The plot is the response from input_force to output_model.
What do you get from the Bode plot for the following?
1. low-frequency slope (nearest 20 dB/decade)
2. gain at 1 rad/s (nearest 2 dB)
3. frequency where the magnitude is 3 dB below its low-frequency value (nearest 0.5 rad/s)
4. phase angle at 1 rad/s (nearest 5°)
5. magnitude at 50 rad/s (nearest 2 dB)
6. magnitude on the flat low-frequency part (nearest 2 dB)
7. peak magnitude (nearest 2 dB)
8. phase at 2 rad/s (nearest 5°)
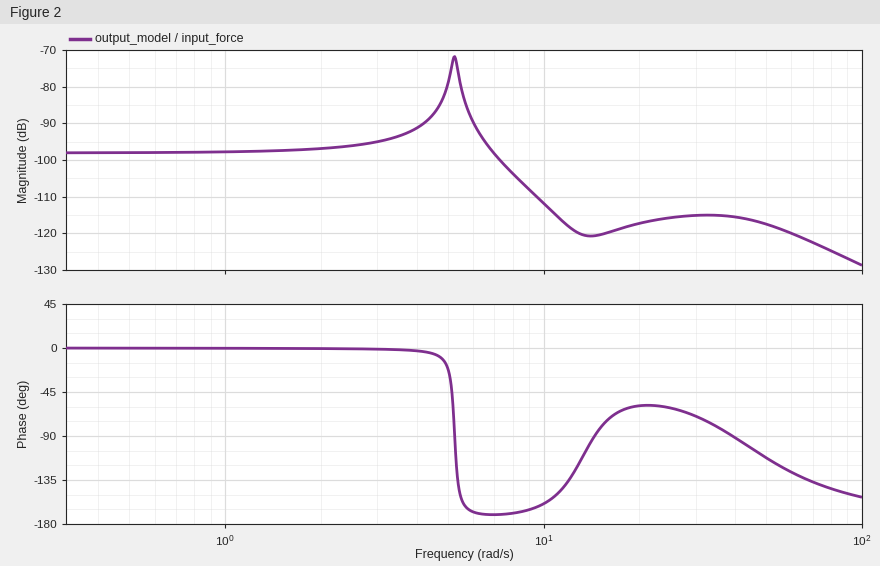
0 dB/decade
-98 dB
7.5 rad/s
0°
-118 dB
-98 dB
-72 dB
0°
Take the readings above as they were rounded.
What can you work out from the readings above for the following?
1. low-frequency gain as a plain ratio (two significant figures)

0.000013
